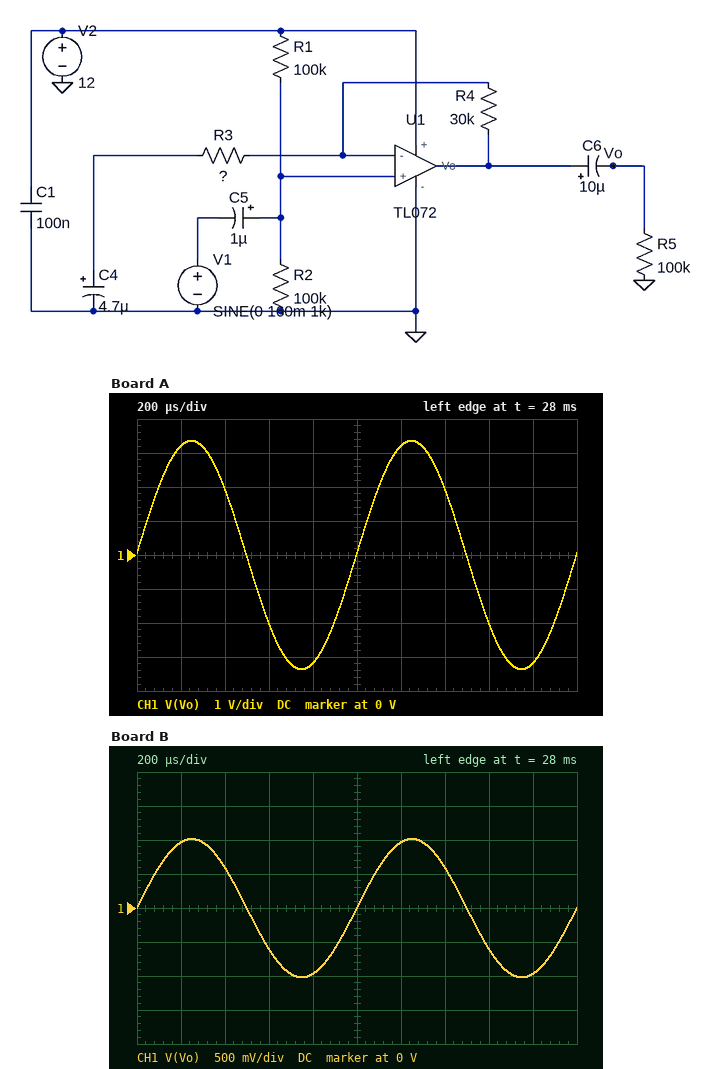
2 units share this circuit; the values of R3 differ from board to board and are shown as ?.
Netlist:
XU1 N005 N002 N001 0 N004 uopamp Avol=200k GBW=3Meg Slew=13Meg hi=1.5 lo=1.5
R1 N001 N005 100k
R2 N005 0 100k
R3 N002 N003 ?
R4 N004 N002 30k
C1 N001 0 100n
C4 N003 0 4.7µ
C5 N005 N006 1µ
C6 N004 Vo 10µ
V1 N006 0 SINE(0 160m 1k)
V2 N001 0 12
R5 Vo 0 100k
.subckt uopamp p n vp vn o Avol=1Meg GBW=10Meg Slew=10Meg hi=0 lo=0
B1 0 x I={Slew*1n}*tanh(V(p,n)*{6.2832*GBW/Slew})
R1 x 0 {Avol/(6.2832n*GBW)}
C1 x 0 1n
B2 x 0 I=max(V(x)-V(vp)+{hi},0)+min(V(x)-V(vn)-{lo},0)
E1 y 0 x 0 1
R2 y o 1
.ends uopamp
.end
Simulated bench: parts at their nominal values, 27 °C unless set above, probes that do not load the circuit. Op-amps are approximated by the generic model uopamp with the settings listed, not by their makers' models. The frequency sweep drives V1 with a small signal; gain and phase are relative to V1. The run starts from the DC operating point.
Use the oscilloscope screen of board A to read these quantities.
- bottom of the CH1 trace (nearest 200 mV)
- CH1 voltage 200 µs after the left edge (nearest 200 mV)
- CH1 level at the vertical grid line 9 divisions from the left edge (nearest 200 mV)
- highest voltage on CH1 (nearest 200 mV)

-3.4 V
3.2 V
-3.2 V
3.4 V
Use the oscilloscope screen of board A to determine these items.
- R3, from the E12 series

1.5 kΩ
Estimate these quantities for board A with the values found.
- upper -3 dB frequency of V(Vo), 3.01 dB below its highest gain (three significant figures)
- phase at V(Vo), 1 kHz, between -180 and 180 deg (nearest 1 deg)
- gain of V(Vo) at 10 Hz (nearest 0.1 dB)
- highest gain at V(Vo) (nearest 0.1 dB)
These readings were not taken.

143 kHz
1 deg
18.2 dB
26.4 dB
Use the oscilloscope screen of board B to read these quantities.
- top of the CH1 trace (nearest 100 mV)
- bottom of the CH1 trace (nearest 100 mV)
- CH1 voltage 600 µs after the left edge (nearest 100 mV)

1.0 V
-1.0 V
-600 mV
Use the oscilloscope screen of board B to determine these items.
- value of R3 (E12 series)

5.6 kΩ
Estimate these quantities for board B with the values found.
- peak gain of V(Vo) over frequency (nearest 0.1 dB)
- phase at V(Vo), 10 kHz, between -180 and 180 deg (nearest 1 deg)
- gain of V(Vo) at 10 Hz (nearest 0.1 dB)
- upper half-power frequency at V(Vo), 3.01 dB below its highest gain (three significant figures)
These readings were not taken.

16.1 dB
-1 deg
14.3 dB
472 kHz
